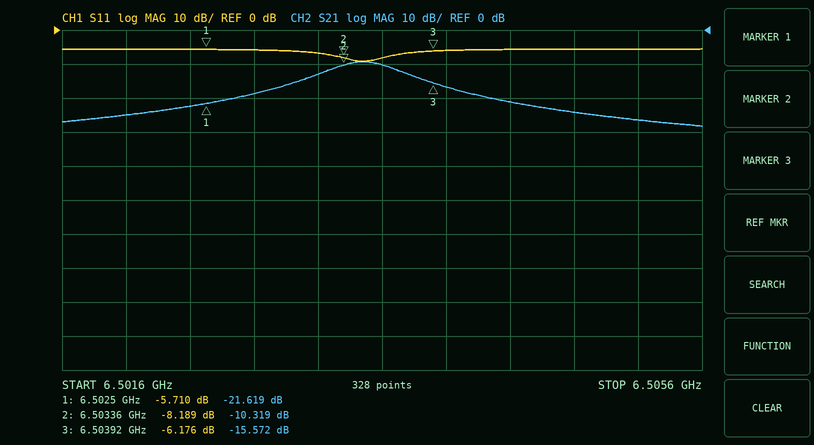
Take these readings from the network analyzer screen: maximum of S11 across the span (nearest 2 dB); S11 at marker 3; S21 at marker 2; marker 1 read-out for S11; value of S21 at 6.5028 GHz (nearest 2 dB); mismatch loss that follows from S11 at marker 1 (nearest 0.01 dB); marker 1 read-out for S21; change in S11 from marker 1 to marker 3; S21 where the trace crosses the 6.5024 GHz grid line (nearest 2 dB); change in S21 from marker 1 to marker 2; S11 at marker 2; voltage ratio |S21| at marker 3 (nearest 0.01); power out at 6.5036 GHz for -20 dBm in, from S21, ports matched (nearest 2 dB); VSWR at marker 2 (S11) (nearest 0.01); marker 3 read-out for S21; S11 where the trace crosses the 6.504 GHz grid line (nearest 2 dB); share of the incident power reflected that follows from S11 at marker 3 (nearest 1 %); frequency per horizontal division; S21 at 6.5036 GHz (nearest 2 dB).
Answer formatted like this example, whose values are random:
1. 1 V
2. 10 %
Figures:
1. -6 dB
2. -6.176 dB
3. -10.319 dB
4. -5.710 dB
5. -18 dB
6. 1.36 dB
7. -21.619 dB
8. -0.466 dB
9. -22 dB
10. 11.300 dB
11. -8.189 dB
12. 0.17
13. -30 dBm
14. 2.28
15. -15.572 dB
16. -6 dB
17. 24 %
18. 400 kHz
19. -10 dB
